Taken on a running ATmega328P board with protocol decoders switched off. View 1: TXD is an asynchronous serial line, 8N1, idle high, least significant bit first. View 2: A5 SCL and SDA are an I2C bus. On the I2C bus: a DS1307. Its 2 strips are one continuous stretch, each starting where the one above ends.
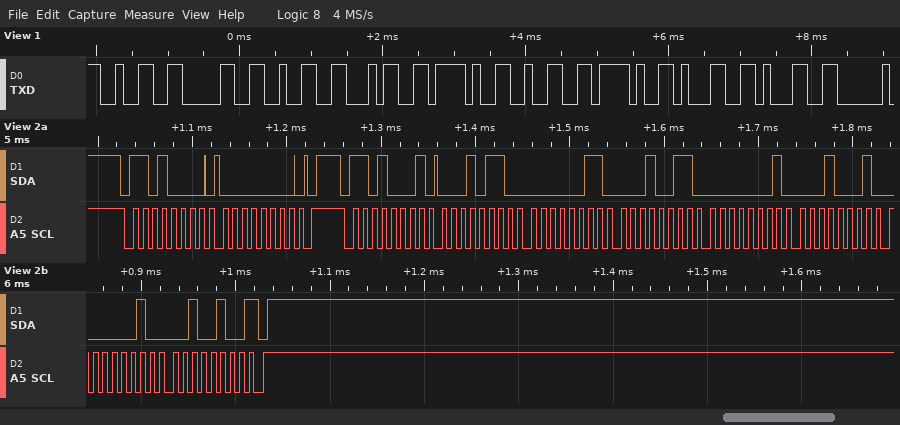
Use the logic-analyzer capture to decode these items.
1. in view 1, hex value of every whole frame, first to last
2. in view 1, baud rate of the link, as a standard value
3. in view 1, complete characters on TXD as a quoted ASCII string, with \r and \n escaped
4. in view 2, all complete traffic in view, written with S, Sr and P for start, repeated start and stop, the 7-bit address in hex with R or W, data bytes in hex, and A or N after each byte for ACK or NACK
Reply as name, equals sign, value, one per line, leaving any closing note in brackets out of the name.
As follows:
in view 1, hex value of every whole frame, first to last = 32 30 32 34 2F 32 2F 31 31
in view 1, baud rate of the link, as a standard value = 9600 baud
in view 1, complete characters on TXD as a quoted ASCII string, with \r and \n escaped = "2024/2/11"
in view 2, all complete traffic in view, written with S, Sr and P for start, repeated start and stop, the 7-bit address in hex with R or W, data bytes in hex, and A or N after each byte for ACK or NACK = S 68W A 00 A P S 68R A 16 A 03 A 13 A 01 A 11 A 02 A 24 N P
